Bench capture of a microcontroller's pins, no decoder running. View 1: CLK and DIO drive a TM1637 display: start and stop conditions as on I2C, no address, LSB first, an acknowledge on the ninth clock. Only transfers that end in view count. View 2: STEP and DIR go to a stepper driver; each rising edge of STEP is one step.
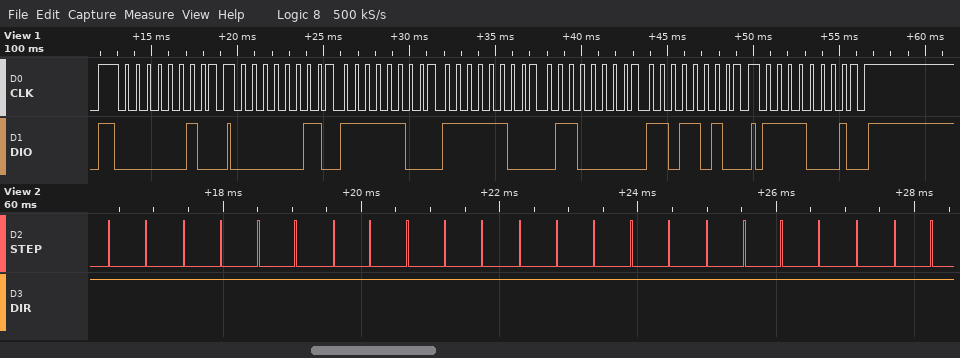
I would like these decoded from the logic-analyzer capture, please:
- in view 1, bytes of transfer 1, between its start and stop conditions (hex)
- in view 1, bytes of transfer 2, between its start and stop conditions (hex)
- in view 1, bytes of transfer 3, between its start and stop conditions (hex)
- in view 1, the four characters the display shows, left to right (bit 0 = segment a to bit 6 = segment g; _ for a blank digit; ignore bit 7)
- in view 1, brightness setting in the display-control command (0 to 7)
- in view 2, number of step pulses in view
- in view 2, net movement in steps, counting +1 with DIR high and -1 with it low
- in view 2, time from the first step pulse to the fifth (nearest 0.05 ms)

40
C0 3F 3F 06 5B
8F
0012
7
23
+23
2.15 ms
